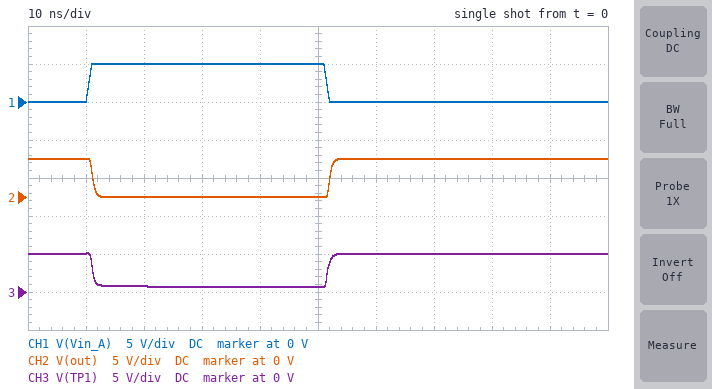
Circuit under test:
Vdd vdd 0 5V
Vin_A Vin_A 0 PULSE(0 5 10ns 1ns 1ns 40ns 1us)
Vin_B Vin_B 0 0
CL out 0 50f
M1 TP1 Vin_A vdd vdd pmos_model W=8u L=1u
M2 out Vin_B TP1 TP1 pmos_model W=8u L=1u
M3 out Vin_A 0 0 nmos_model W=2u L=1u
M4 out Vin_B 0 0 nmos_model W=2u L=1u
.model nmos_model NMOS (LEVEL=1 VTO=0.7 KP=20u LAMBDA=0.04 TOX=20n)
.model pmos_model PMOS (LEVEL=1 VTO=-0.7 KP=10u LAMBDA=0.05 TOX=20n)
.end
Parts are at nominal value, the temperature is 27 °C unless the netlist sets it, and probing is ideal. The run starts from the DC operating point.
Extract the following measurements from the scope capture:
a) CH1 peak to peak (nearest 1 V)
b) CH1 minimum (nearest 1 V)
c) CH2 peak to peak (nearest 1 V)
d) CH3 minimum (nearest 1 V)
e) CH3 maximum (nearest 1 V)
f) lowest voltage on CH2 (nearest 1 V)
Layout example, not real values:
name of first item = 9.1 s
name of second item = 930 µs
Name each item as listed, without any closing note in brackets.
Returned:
CH1 peak to peak = 5 V
CH1 minimum = 0 V
CH2 peak to peak = 5 V
CH3 minimum = 1 V
CH3 maximum = 5 V
lowest voltage on CH2 = 0 V
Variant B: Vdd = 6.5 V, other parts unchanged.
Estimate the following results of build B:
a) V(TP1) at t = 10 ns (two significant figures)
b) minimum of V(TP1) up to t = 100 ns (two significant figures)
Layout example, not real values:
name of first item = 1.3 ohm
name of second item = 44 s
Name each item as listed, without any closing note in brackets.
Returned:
V(TP1) at t = 10 ns = 6.5 V
minimum of V(TP1) up to t = 100 ns = 1.6 V
